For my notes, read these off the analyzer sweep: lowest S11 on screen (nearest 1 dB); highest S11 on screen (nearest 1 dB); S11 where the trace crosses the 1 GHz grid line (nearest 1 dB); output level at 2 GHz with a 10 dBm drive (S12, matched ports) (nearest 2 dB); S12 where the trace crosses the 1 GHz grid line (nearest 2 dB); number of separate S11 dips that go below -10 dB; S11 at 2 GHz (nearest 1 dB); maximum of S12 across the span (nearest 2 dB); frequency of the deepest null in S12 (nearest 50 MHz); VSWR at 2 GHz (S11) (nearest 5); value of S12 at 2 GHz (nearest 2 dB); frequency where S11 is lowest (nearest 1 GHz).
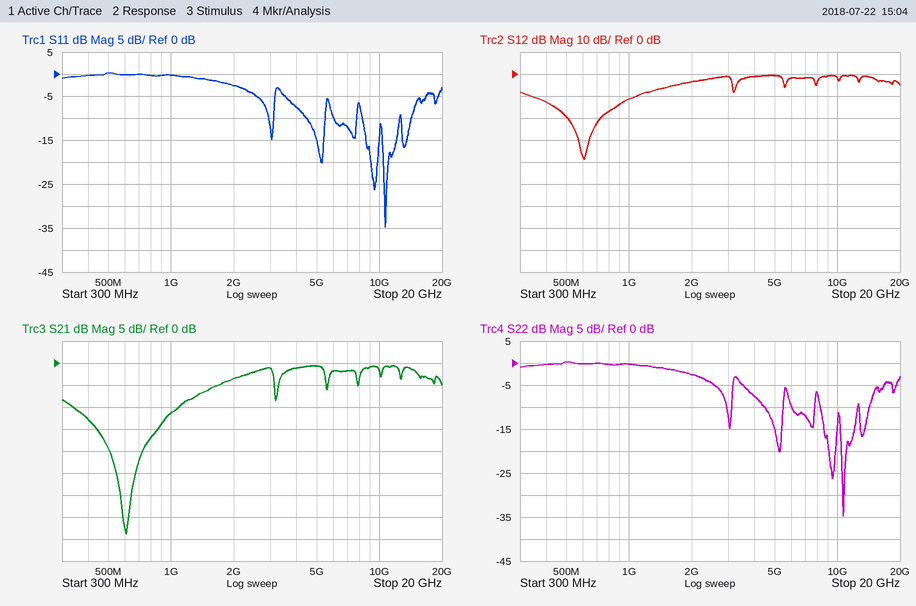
-35 dB
0 dB
0 dB
6 dBm
-12 dB
6
-3 dB
0 dB
600 MHz
5
-4 dB
11 GHz
